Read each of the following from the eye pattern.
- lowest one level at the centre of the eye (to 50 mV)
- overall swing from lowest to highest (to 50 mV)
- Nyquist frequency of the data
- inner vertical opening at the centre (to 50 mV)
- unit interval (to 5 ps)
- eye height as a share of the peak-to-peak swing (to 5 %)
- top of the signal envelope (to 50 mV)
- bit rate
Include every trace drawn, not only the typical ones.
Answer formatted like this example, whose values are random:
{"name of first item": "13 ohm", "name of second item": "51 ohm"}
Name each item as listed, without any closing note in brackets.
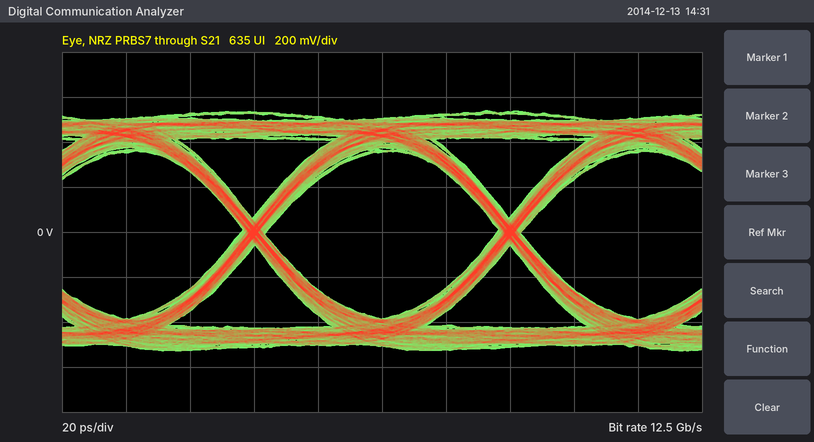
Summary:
{"lowest one level at the centre of the eye": "350 mV", "overall swing from lowest to highest": "1.05 V", "Nyquist frequency of the data": "6.25 GHz", "inner vertical opening at the centre": "750 mV", "unit interval": "80 ps", "eye height as a share of the peak-to-peak swing": "70 %", "top of the signal envelope": "550 mV", "bit rate": "12.5 Gb/s"}
